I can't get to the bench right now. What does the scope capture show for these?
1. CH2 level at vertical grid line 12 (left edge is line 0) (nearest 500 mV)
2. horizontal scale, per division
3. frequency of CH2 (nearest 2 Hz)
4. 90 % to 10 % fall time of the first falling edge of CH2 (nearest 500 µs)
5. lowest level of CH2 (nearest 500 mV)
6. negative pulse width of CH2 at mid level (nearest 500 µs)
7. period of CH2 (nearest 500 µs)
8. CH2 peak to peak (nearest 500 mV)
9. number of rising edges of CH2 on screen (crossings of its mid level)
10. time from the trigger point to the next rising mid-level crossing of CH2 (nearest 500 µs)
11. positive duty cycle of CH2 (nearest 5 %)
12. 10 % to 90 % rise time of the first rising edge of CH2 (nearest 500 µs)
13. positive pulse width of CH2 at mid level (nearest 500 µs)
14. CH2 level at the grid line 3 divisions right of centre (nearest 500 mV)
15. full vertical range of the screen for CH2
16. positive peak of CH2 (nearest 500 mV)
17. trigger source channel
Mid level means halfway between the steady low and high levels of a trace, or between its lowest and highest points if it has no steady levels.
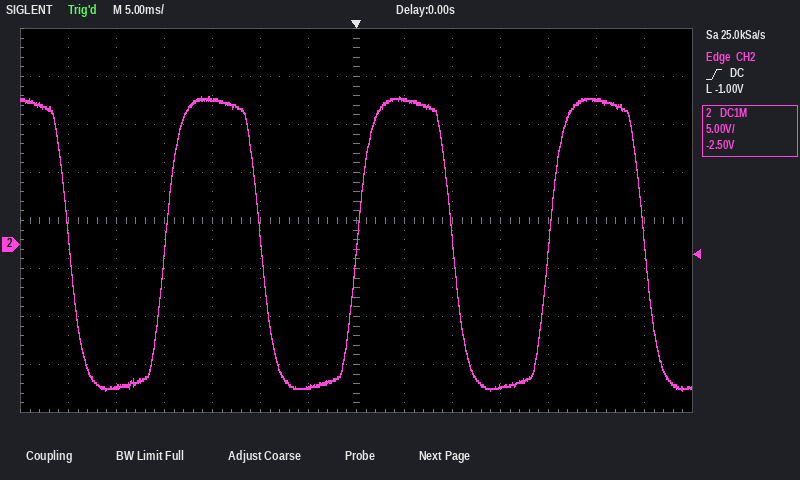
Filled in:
15.0 V
5 ms
50 Hz
3.0 ms
-15.0 V
10.0 ms
20.0 ms
30.5 V
3
20.0 ms
50 %
3.0 ms
10.0 ms
-15.0 V
40 V
15.5 V
CH2
